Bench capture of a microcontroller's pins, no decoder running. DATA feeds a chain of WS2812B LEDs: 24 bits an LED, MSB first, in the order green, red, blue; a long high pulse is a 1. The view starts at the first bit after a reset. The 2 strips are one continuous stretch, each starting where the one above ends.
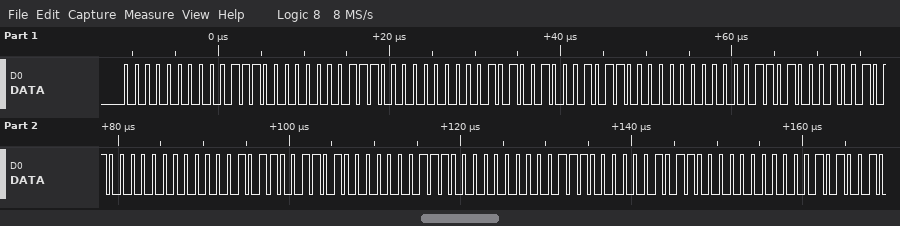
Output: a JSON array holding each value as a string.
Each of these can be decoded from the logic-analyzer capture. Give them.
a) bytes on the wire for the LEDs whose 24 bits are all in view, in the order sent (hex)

["00 38 07 00 29 16 00 1A 25 00 0B 34 07 00 38 16 00 29"]
